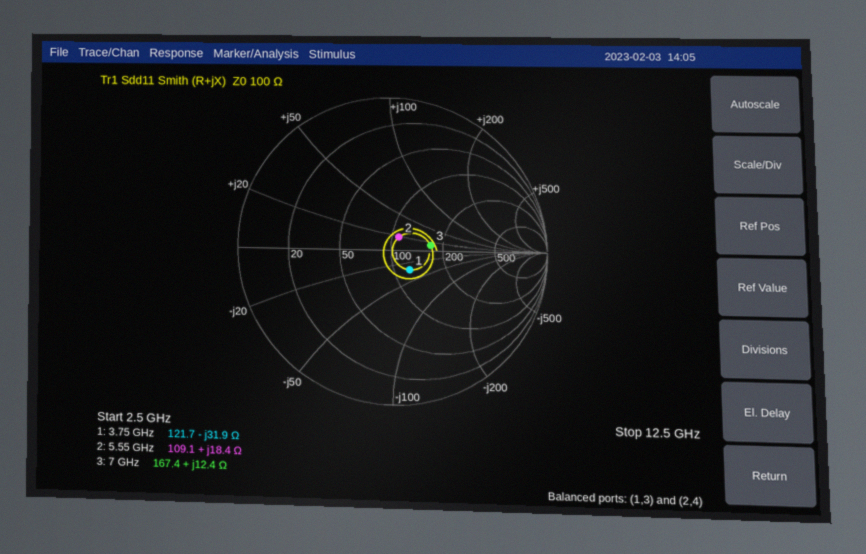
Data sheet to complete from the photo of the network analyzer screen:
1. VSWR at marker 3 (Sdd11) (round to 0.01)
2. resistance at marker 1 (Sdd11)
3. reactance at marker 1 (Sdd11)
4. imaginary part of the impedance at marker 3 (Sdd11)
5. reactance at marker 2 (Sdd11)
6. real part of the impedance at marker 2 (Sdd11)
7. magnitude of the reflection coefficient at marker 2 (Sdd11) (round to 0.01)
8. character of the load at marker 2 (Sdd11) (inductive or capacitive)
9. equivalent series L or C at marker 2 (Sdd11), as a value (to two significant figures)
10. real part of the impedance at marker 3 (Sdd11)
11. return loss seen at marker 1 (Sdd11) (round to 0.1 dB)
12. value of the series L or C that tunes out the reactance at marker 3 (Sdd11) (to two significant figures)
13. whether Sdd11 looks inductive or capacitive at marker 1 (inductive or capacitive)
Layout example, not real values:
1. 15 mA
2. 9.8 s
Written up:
1. 1.69
2. 121.7 Ω
3. -31.9 Ω
4. +12.4 Ω
5. +18.4 Ω
6. 109.1 Ω
7. 0.10
8. inductive
9. 530 pH
10. 167.4 Ω
11. 15.3 dB
12. 1.8 pF
13. capacitive
